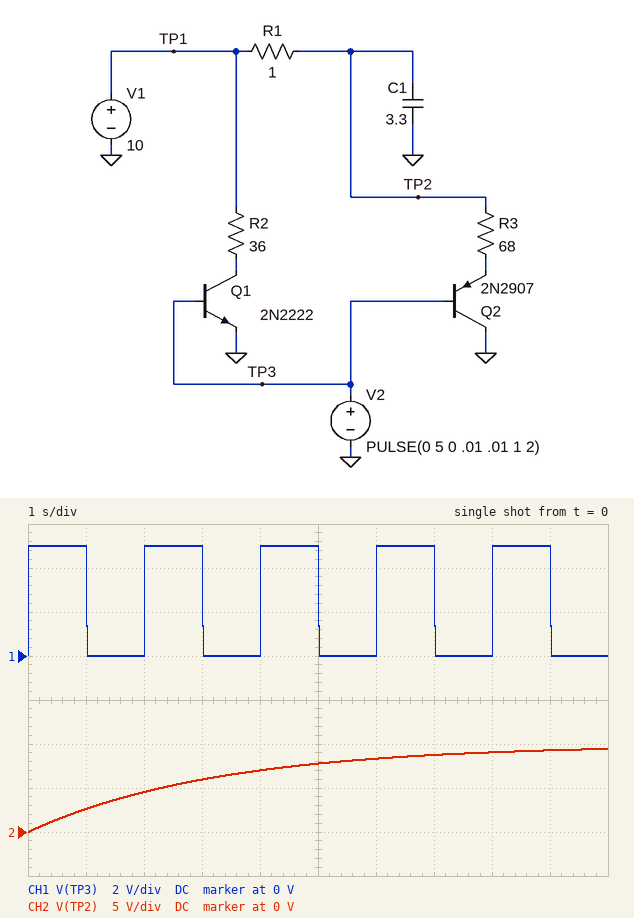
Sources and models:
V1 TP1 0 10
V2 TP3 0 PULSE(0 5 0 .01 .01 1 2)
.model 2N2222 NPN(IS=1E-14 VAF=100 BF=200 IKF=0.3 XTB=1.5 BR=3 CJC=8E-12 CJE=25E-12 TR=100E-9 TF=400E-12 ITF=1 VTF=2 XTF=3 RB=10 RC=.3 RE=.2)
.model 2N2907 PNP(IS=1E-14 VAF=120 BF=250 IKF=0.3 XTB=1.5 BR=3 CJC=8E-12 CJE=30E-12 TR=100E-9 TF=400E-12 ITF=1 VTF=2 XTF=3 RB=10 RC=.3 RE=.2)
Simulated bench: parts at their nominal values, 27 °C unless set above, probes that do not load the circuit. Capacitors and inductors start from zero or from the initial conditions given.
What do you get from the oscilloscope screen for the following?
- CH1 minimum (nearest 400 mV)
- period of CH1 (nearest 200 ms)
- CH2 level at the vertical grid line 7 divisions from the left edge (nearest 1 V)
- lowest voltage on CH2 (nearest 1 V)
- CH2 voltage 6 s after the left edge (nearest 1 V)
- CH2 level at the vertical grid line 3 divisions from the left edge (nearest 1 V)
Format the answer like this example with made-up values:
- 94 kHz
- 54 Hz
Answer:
- 0 V
- 2.0 s
- 9 V
- 0 V
- 8 V
- 6 V
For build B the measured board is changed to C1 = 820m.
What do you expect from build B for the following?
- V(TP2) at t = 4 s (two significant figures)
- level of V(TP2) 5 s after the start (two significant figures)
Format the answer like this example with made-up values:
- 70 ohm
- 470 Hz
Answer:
- 9.8 V
- 9.9 V
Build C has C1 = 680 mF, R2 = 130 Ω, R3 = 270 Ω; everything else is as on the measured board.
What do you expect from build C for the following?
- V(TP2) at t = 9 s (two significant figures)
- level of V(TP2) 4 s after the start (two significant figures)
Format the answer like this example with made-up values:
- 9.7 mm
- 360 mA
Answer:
- 10 V
- 9.9 V
